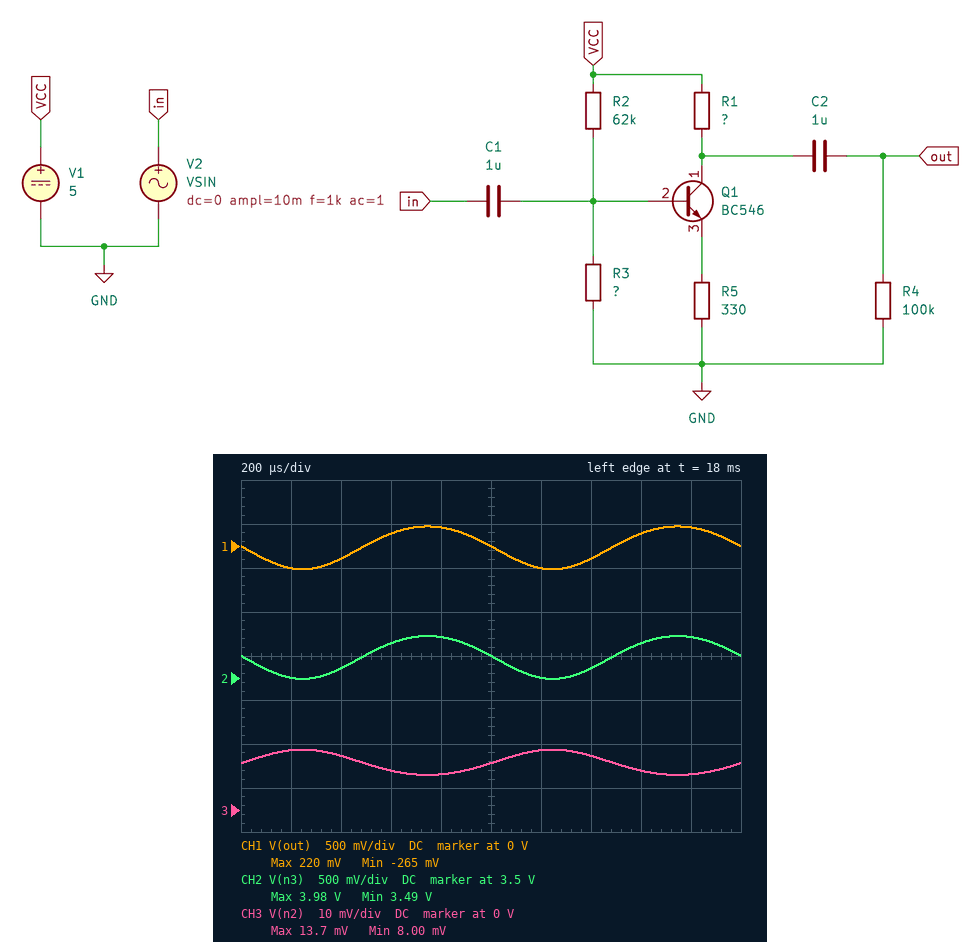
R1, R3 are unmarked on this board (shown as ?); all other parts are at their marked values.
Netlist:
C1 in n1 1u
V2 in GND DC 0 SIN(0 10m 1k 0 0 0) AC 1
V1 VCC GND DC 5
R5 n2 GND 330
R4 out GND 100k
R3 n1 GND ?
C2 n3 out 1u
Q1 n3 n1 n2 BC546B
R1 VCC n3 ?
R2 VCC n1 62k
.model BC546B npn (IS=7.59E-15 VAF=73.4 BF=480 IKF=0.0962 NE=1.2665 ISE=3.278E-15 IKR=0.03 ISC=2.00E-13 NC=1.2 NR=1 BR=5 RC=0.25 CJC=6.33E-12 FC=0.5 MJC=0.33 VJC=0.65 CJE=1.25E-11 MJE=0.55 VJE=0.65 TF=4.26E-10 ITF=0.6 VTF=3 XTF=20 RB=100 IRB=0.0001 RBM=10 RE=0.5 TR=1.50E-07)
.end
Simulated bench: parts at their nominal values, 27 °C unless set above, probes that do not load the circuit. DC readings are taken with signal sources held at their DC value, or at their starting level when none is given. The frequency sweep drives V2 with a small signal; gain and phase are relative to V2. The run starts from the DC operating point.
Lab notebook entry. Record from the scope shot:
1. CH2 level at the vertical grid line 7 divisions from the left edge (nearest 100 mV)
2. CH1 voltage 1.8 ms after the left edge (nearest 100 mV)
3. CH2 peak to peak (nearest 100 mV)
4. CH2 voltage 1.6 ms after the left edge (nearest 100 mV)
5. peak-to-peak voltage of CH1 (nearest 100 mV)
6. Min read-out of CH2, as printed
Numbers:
3.6 V
200 mV
500 mV
3.9 V
500 mV
3.49 V
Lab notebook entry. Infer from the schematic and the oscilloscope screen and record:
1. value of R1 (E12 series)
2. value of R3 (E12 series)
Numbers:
39 kΩ
8.2 kΩ
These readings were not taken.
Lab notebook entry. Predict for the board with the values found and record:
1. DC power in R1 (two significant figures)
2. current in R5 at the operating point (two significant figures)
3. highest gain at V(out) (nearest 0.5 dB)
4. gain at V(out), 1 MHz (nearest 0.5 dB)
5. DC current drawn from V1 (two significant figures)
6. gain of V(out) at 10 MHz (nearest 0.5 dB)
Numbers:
40 µW
32 µA
27.5 dB
26.0 dB
100 µA
11.0 dB
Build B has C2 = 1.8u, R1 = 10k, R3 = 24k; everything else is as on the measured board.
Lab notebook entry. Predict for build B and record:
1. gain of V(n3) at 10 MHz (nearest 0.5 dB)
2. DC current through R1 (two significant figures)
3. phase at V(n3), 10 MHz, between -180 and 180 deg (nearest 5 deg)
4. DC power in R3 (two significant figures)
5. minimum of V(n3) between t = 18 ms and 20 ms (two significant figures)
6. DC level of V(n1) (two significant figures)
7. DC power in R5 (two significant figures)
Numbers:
-1.5 dB
480 µA
10 deg
28 µW
230 mV
820 mV
86 µW
